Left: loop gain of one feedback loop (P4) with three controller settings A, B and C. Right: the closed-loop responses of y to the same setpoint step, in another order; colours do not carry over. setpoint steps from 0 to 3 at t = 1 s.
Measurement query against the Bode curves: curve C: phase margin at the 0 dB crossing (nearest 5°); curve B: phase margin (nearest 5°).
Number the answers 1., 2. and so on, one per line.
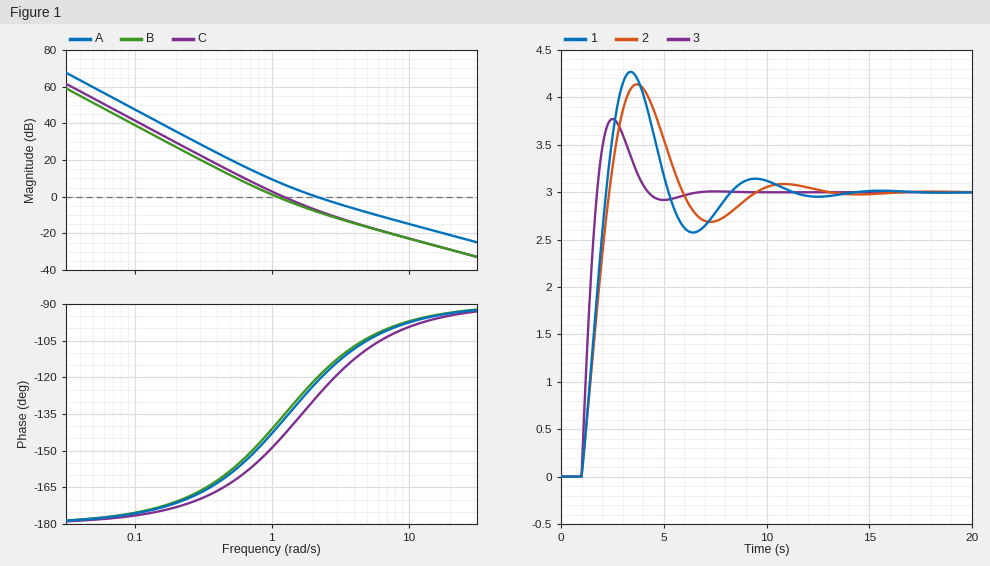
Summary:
1. 35°
2. 40°
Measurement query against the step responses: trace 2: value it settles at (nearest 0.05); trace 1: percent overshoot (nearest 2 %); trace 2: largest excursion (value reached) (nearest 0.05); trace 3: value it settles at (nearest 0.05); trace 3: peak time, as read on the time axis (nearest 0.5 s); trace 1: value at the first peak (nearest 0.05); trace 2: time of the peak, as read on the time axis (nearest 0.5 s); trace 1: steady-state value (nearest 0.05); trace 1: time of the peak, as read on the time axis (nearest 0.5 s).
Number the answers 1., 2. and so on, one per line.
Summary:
1. 3.00
2. 42 %
3. 4.15
4. 3.00
5. 2.5 s
6. 4.25
7. 3.5 s
8. 3.00
9. 3.5 s
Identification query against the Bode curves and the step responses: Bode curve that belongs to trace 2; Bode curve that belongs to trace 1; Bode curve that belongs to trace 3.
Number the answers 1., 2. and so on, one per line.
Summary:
1. B
2. C
3. A
